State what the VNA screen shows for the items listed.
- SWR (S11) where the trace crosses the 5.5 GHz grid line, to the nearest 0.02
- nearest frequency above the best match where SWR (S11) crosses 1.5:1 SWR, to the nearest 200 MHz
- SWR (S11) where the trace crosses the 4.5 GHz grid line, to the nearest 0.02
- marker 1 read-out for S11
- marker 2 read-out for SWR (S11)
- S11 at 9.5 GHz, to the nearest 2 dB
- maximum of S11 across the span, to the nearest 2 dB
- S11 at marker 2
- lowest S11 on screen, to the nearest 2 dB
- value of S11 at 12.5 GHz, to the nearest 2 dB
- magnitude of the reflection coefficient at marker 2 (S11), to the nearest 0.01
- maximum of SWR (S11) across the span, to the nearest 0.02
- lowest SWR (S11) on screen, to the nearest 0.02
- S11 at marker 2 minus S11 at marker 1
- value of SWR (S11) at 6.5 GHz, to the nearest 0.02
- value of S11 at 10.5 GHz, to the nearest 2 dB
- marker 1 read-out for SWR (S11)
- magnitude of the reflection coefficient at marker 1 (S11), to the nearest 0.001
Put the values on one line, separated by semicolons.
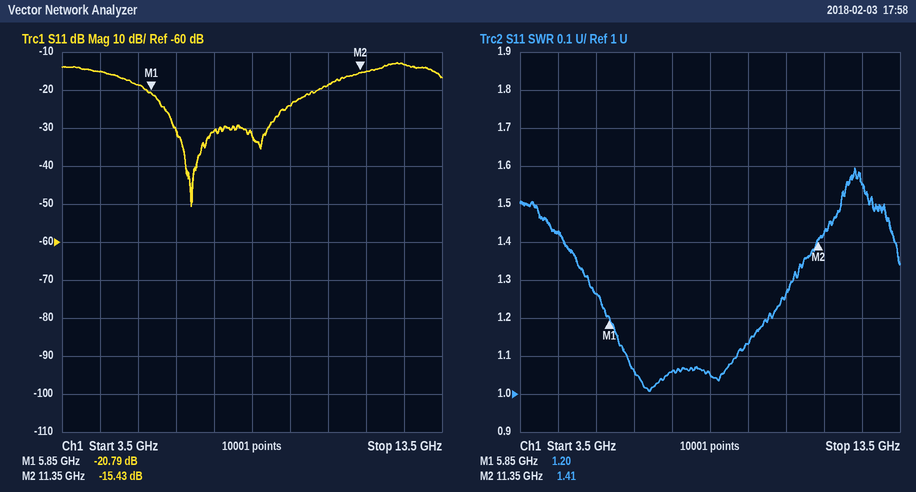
1.26; 12.0 GHz; 1.42; -20.79 dB; 1.41; -24 dB; -12 dB; -15.43 dB; -50 dB; -14 dB; 0.17; 1.60; 1.00; 5.36 dB; 1.06; -18 dB; 1.20; 0.091
